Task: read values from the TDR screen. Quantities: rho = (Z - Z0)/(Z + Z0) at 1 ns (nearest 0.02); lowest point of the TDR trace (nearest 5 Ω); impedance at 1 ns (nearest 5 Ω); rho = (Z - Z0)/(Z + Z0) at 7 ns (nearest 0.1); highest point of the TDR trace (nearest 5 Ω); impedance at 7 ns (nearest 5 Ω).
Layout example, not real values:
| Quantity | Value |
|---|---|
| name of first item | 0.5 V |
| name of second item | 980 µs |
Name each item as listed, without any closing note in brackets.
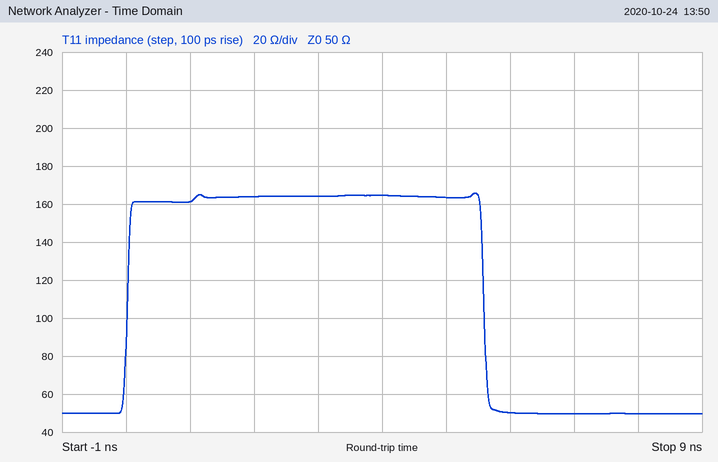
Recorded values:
| Quantity | Value |
|---|---|
| rho = (Z - Z0)/(Z + Z0) at 1 ns | +0.52 |
| lowest point of the TDR trace | 50 Ω |
| impedance at 1 ns | 160 Ω |
| rho = (Z - Z0)/(Z + Z0) at 7 ns | 0.0 |
| highest point of the TDR trace | 165 Ω |
| impedance at 7 ns | 50 Ω |
